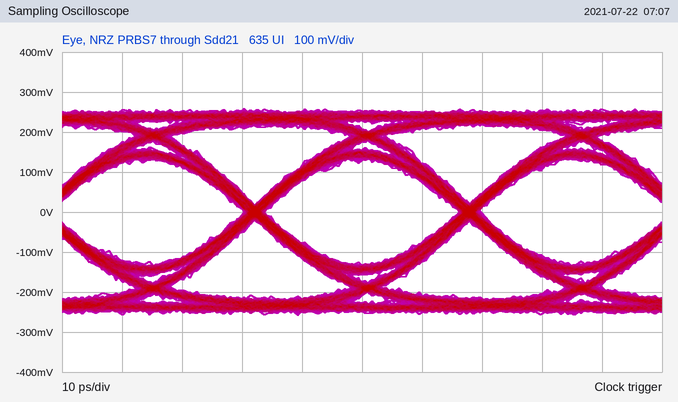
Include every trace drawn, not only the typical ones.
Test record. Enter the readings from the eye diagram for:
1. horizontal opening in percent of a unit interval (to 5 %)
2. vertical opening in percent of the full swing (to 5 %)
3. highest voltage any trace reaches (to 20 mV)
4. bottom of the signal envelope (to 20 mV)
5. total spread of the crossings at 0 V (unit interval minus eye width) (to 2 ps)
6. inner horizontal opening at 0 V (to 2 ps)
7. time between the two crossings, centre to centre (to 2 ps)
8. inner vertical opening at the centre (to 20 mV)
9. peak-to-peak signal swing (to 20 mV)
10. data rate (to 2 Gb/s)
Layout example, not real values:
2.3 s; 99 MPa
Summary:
90 %; 50 %; 260 mV; -260 mV; 4 ps; 32 ps; 36 ps; 260 mV; 520 mV; 28 Gb/s
